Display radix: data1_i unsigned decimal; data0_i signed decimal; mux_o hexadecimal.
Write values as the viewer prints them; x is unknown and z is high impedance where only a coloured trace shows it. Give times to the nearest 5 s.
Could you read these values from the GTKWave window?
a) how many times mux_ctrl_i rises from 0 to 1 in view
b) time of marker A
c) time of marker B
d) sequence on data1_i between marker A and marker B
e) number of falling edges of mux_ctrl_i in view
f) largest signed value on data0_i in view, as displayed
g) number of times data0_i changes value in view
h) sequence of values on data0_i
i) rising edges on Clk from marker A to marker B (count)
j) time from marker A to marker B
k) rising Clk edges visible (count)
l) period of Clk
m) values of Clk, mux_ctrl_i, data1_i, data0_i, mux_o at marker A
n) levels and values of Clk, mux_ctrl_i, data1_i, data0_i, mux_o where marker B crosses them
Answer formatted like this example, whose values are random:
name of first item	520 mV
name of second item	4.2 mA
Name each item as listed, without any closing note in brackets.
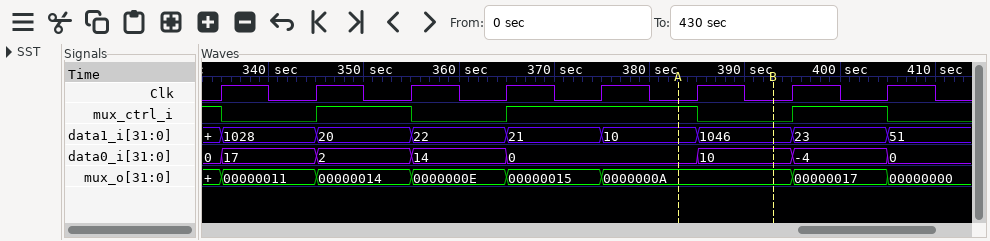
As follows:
how many times mux_ctrl_i rises from 0 to 1 in view	3
time of marker A	385 s
time of marker B	395 s
sequence on data1_i between marker A and marker B	10, 1046
number of falling edges of mux_ctrl_i in view	4
largest signed value on data0_i in view, as displayed	17
number of times data0_i changes value in view	7
sequence of values on data0_i	0, 17, 2, 14, 0, 10, -4, 0
rising edges on Clk from marker A to marker B	1
time from marker A to marker B	10 s
rising Clk edges visible	8
period of Clk	10 s
values of Clk, mux_ctrl_i, data1_i, data0_i, mux_o at marker A	Clk=0, mux_ctrl_i=1, data1_i=10, data0_i=0, mux_o=0000000A
levels and values of Clk, mux_ctrl_i, data1_i, data0_i, mux_o where marker B crosses them	Clk=0, mux_ctrl_i=0, data1_i=1046, data0_i=10, mux_o=0000000A
